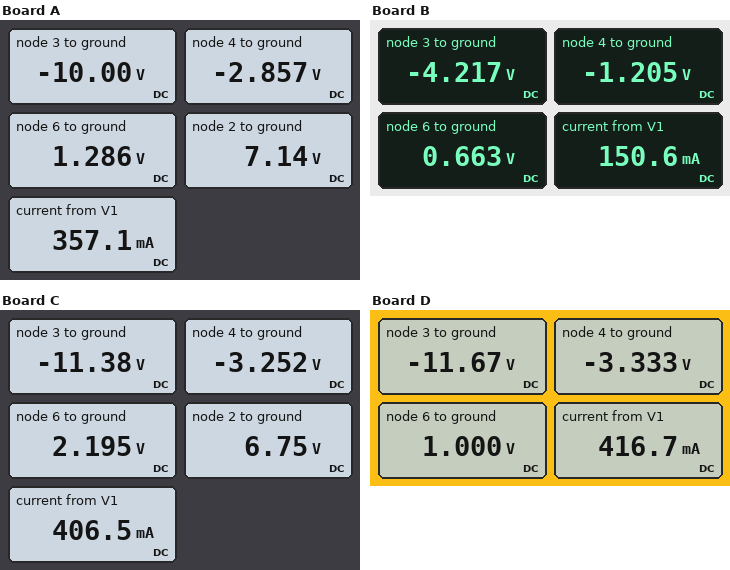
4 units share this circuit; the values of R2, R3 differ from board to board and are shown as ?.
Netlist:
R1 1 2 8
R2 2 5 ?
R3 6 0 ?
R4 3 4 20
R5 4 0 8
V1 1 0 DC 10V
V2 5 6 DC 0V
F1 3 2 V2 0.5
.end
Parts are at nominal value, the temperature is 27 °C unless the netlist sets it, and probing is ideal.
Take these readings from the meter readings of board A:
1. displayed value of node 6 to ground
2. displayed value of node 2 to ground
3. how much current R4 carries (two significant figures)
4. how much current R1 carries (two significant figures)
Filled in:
1.286 V
7.14 V
360 mA
360 mA
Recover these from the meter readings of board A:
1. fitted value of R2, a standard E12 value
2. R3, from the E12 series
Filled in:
8.2 Ω
1.8 Ω
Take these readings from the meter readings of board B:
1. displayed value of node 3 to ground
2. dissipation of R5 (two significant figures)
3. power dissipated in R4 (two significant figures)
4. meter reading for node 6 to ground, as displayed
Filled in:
-4.217 V
180 mW
450 mW
0.663 V
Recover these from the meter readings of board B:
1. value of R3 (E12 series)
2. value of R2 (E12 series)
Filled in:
2.2 Ω
27 Ω
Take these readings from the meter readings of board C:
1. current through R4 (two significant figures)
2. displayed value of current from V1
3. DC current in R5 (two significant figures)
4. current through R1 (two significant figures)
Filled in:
410 mA
406.5 mA
410 mA
410 mA
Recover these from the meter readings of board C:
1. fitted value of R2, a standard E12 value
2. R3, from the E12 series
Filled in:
5.6 Ω
2.7 Ω
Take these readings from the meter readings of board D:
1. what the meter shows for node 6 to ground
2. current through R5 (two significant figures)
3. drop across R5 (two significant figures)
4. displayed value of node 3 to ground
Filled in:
1.000 V
420 mA
3.3 V
-11.67 V
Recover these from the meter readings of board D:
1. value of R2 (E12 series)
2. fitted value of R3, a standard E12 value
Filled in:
6.8 Ω
1.2 Ω
